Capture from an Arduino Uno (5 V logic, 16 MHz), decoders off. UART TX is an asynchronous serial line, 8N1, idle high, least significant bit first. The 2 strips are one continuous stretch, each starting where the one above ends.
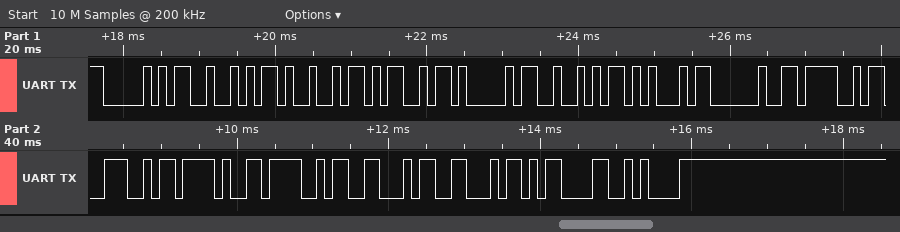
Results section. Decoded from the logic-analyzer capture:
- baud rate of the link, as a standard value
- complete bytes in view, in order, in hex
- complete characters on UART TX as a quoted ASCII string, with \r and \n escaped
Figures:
9600 baud
50 52 49 4D 41 52 45 20 4F 4E 2F 4F 46 46 0D 0A
"PRIMARE ON/OFF\r\n"
